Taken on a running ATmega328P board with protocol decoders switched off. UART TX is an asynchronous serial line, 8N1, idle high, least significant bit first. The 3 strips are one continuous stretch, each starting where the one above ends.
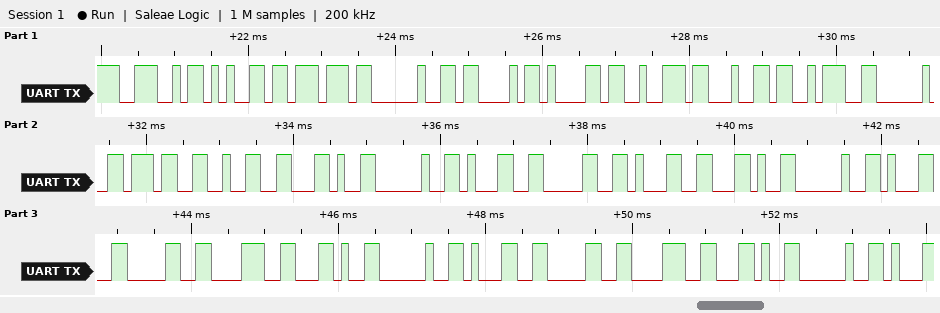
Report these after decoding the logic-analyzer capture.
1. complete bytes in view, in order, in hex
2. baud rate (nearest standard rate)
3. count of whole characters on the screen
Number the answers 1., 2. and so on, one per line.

1. 4E 65 77 20 43 61 72 64 3A 20 37 32 2C 20 31 30 31 2C 20 31 30 38 2C 20 31 30 38 2C 20
2. 9600 baud
3. 29
